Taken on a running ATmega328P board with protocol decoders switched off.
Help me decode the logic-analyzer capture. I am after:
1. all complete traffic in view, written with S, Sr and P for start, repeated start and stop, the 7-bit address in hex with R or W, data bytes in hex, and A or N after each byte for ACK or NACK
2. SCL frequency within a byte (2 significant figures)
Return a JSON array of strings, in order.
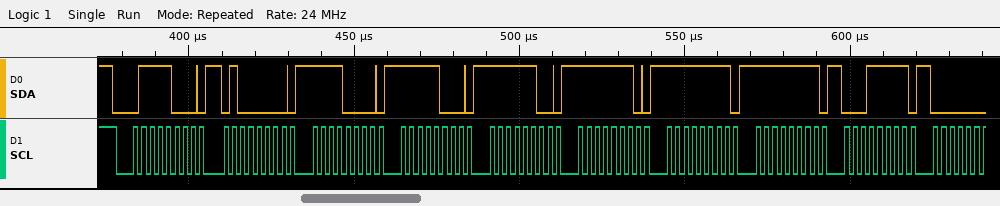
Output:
["S 3CW A 40 A F0 A F8 A FC A FE A FF A FF A 1F A", "400 kHz"]
